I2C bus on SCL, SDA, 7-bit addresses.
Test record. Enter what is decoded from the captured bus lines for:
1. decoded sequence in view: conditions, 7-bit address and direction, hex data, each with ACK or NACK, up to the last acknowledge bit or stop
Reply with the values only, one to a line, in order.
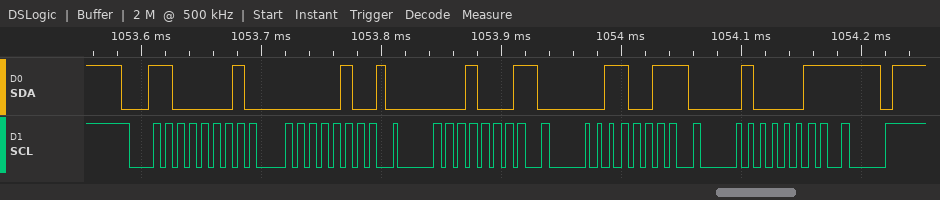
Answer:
start, address 60 read ACK, 04 ACK, 11 ACK, 33 ACK, 43 NACK, stop
